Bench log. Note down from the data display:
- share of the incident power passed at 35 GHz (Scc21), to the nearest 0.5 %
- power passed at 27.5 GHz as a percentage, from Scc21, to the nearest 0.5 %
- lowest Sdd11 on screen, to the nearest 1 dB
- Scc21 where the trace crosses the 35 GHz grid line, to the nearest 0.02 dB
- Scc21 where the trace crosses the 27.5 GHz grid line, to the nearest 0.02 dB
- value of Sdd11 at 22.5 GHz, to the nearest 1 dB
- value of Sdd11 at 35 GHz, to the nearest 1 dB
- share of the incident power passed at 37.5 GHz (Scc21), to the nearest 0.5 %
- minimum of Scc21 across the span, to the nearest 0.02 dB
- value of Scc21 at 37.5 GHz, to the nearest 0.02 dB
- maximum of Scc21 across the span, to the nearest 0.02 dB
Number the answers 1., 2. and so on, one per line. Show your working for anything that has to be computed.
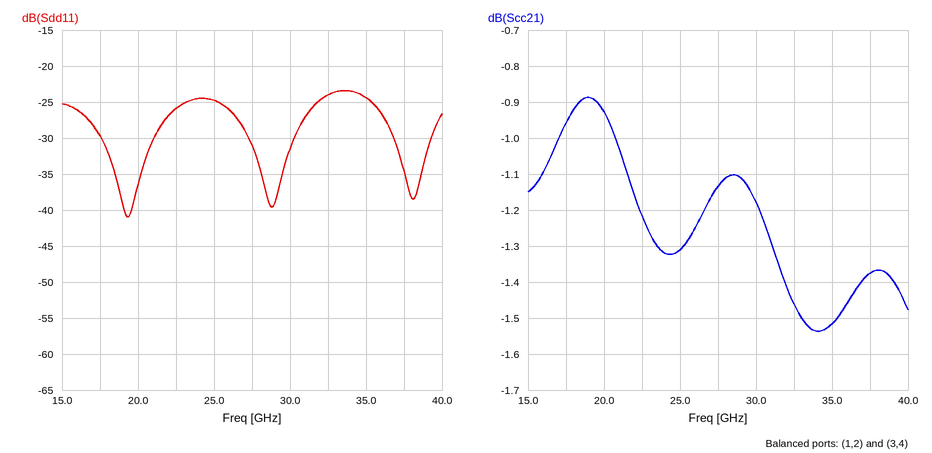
1. 10^(-1.52/10) ≈ 70.5 %
2. 10^(-1.14/10) ≈ 76.9 %, so 77.0 % to the nearest 0.5 %
3. -41 dB
4. -1.52 dB
5. -1.14 dB
6. -26 dB
7. -24 dB
8. 10^(-1.38/10) ≈ 72.8 %, so 73.0 % to the nearest 0.5 %
9. -1.54 dB
10. -1.38 dB
11. -0.88 dB
